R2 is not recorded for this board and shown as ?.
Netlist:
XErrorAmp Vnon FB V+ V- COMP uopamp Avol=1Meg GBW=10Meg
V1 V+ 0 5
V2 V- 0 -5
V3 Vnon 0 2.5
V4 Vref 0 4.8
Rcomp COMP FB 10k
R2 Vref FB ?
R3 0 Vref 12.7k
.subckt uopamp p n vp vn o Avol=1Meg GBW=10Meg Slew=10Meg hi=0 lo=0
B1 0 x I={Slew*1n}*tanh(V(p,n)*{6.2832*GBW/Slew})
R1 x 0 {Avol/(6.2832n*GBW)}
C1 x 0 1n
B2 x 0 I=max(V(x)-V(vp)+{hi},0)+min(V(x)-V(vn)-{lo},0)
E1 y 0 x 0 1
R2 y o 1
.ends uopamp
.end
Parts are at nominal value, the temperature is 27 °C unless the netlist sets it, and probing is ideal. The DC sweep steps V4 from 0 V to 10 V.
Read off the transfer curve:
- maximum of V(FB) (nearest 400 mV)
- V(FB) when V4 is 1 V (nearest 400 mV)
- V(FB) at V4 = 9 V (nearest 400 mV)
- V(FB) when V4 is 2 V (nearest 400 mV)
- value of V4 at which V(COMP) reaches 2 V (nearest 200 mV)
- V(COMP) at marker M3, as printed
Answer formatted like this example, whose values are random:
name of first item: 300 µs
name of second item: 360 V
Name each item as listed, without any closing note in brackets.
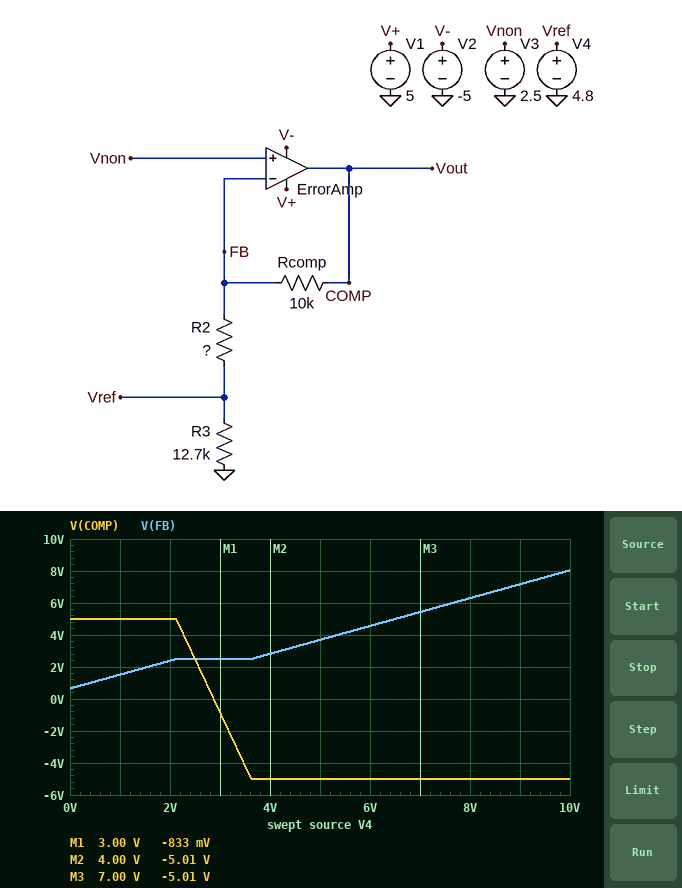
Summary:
maximum of V(FB): 8.0 V
V(FB) when V4 is 1 V: 1.6 V
V(FB) at V4 = 9 V: 7.2 V
V(FB) when V4 is 2 V: 2.4 V
value of V4 at which V(COMP) reaches 2 V: 2.6 V
V(COMP) at marker M3, as printed: -5.01 V
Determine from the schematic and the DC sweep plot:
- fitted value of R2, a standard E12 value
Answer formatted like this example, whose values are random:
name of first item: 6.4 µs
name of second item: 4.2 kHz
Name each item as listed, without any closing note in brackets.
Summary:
fitted value of R2, a standard E12 value: 1.5 kΩ
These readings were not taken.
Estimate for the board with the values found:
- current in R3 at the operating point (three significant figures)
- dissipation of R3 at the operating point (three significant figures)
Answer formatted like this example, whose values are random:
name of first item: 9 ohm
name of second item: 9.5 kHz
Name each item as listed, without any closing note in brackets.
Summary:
current in R3 at the operating point: 378 µA
dissipation of R3 at the operating point: 1.81 mW
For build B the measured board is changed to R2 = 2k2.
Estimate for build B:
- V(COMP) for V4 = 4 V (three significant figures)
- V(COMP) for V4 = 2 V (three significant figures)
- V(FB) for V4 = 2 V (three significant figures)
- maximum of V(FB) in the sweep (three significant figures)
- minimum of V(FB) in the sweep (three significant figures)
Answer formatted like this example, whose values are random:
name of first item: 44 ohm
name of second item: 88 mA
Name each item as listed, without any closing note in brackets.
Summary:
V(COMP) for V4 = 4 V: -4.32 V
V(COMP) for V4 = 2 V: 4.77 V
V(FB) for V4 = 2 V: 2.50 V
maximum of V(FB) in the sweep: 7.29 V
minimum of V(FB) in the sweep: 903 mV
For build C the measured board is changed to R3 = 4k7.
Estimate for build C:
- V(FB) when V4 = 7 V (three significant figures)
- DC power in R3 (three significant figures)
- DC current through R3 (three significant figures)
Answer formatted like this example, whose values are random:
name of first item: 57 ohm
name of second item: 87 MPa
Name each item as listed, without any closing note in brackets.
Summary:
V(FB) when V4 = 7 V: 5.43 V
DC power in R3: 4.90 mW
DC current through R3: 1.02 mA
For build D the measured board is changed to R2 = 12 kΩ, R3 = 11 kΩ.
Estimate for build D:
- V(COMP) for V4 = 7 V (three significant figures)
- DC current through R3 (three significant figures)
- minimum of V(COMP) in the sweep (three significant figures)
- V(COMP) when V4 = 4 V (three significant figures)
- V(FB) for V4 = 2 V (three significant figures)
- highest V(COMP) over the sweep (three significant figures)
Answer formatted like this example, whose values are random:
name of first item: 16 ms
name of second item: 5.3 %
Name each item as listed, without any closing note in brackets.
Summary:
V(COMP) for V4 = 7 V: -1.25 V
DC current through R3: 436 µA
minimum of V(COMP) in the sweep: -3.75 V
V(COMP) when V4 = 4 V: 1.25 V
V(FB) for V4 = 2 V: 2.50 V
highest V(COMP) over the sweep: 4.58 V
